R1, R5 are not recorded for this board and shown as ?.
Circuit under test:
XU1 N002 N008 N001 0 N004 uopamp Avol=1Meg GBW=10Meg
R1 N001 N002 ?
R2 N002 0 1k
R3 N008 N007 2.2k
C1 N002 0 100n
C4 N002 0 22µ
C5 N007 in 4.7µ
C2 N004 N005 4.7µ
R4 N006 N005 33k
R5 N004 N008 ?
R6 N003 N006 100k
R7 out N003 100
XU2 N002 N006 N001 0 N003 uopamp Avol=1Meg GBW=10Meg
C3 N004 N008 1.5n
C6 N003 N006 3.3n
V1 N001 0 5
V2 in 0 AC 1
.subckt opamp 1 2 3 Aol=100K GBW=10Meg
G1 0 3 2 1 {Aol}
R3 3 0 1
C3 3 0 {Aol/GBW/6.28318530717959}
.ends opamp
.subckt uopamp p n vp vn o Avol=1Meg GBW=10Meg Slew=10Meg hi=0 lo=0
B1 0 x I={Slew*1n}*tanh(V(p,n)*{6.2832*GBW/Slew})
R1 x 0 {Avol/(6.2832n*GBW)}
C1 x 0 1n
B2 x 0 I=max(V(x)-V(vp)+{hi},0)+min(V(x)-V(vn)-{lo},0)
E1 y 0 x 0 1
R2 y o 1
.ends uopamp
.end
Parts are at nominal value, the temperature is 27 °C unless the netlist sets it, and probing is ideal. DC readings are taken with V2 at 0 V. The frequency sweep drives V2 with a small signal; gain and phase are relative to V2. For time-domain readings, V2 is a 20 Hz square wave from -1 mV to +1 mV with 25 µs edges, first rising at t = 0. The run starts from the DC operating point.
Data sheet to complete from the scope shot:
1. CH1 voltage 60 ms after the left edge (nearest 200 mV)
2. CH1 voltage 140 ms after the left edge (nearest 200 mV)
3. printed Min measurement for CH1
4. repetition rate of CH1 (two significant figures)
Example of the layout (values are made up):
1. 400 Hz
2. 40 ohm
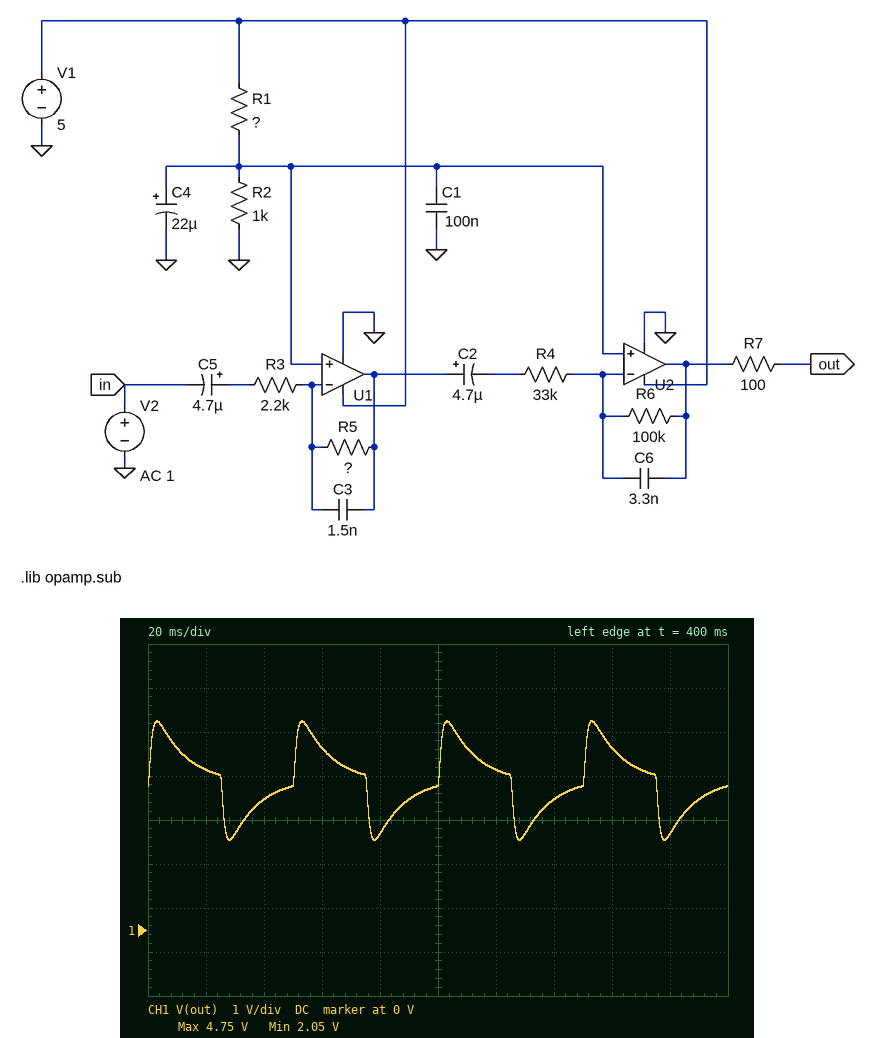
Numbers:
1. 4.2 V
2. 3.0 V
3. 2.05 V
4. 20 Hz
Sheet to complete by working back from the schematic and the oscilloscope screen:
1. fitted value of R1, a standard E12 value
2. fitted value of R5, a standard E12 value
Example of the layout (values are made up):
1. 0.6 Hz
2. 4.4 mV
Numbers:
1. 470 Ω
2. 680 kΩ
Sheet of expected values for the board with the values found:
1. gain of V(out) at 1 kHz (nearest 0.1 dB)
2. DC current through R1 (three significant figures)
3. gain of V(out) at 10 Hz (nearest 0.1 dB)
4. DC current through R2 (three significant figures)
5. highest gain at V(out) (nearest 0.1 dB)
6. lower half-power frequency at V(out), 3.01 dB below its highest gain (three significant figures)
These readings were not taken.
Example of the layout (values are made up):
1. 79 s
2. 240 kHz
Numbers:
1. 35.9 dB
2. 3.40 mA
3. 54.1 dB
4. 3.40 mA
5. 58.6 dB
6. 13.0 Hz
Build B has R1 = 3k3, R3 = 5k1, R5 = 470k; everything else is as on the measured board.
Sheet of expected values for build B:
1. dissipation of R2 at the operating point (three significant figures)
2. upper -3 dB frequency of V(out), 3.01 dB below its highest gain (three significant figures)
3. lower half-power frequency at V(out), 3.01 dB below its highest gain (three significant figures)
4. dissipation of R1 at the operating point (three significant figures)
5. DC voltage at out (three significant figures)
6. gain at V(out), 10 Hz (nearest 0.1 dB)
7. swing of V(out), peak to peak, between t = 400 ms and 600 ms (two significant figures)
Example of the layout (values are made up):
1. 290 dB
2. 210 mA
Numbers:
1. 1.35 mW
2. 203 Hz
3. 6.39 Hz
4. 4.46 mW
5. 1.16 V
6. 47.3 dB
7. 760 mV
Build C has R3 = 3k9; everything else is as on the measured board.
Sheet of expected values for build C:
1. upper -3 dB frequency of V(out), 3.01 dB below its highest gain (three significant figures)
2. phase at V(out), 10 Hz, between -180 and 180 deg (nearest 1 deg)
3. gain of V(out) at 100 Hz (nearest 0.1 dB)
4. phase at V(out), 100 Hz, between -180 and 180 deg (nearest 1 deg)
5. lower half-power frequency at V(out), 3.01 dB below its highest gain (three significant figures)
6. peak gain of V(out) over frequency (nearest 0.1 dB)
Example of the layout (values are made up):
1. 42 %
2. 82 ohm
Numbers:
1. 157 Hz
2. 42 deg
3. 52.7 dB
4. -39 deg
5. 7.92 Hz
6. 54.0 dB
